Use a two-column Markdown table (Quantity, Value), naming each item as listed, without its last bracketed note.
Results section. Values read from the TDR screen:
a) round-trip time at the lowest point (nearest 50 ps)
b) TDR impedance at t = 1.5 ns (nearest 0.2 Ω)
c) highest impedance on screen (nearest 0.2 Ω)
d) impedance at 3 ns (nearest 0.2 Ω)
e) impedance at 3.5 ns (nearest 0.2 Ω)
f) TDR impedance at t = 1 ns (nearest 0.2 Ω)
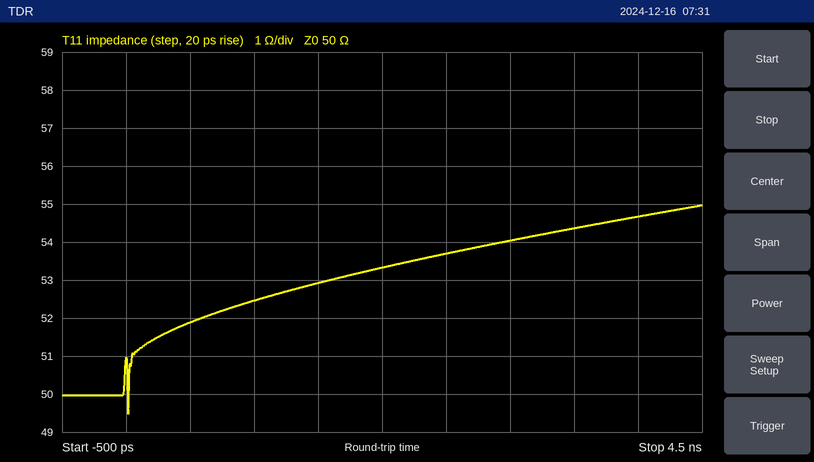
| Quantity | Value |
|---|---|
| round-trip time at the lowest point | 0 ps |
| TDR impedance at t = 1.5 ns | 53.0 Ω |
| highest impedance on screen | 55.0 Ω |
| impedance at 3 ns | 54.0 Ω |
| impedance at 3.5 ns | 54.4 Ω |
| TDR impedance at t = 1 ns | 52.4 Ω |
